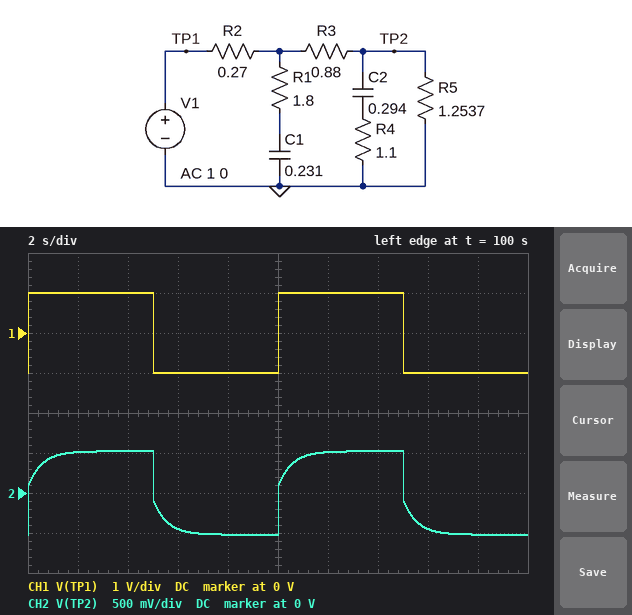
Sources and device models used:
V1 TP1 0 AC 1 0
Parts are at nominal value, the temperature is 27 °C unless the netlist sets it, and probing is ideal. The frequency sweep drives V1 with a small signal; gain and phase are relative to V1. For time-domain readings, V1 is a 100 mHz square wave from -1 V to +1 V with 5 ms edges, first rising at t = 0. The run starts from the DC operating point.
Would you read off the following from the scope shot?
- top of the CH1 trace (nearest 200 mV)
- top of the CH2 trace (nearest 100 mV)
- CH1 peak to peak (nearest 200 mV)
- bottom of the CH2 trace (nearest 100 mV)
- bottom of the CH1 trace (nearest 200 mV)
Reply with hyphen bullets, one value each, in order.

- 1.0 V
- 500 mV
- 2.0 V
- -500 mV
- -1.0 V
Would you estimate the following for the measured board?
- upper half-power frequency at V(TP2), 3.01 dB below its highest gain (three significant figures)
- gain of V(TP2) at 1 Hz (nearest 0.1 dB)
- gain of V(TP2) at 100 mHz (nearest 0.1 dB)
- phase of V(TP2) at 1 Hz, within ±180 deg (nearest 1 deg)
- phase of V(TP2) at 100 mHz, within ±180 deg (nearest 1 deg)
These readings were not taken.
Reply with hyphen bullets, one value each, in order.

- 498 mHz
- -9.8 dB
- -6.0 dB
- -11 deg
- -8 deg
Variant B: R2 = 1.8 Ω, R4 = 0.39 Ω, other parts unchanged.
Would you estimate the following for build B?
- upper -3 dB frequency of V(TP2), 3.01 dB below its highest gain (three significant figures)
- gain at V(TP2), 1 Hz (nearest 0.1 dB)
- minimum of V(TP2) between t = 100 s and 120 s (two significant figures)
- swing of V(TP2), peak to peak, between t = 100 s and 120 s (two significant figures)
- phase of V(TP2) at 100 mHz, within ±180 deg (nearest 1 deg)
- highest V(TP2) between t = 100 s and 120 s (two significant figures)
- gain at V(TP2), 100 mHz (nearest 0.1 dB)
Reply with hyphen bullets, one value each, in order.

- 274 mHz
- -18.9 dB
- -320 mV
- 640 mV
- -16 deg
- 320 mV
- -10.6 dB
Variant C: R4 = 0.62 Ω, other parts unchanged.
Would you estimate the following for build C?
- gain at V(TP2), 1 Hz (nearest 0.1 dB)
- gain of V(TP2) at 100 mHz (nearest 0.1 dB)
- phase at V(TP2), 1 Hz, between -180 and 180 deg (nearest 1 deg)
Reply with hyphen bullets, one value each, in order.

- -10.8 dB
- -5.9 dB
- -19 deg
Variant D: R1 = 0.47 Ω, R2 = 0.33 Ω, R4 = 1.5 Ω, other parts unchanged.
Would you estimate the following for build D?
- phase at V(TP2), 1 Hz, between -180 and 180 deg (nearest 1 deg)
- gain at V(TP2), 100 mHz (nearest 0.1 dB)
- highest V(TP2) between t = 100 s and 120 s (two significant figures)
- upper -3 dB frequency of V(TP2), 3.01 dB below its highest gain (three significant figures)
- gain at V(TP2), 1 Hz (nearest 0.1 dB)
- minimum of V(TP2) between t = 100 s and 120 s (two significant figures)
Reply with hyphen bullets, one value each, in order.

- -18 deg
- -6.2 dB
- 510 mV
- 540 mHz
- -10.3 dB
- -510 mV
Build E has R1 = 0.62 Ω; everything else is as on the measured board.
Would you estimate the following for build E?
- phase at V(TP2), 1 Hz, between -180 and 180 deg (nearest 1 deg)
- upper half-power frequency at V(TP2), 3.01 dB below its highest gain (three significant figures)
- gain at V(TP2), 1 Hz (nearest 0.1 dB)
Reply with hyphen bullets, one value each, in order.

- -17 deg
- 512 mHz
- -10.4 dB
